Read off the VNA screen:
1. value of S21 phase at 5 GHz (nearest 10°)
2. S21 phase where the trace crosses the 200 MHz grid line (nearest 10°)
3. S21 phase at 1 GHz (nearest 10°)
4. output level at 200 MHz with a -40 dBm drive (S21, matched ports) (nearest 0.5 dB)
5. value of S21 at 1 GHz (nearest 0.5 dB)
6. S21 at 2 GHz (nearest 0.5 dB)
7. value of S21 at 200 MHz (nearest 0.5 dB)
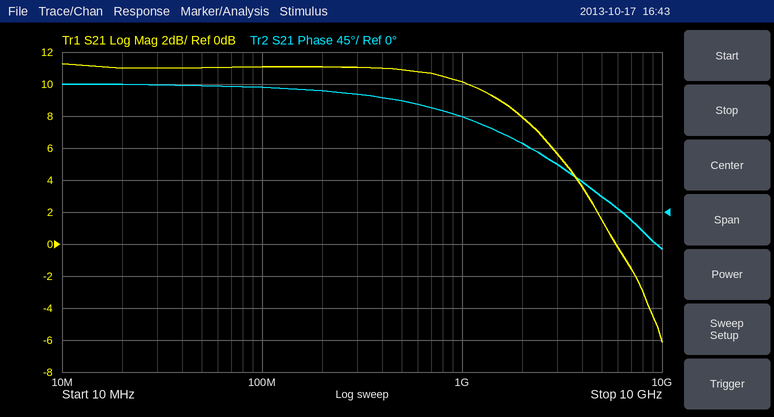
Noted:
20°
170°
130°
-29.0 dBm
10.0 dB
8.0 dB
11.0 dB
